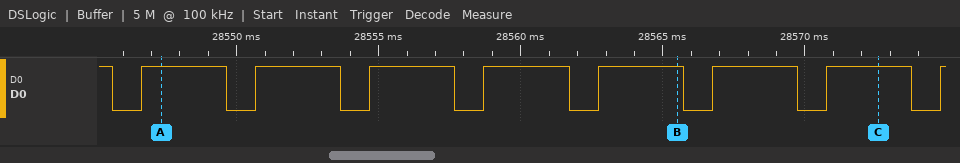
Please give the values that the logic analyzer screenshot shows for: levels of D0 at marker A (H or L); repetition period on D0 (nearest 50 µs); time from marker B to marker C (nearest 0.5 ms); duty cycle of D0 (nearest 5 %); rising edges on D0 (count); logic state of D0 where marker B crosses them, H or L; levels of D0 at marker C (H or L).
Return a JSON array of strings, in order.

["D0=H", "4000 µs", "7 ms", "75 %", "8", "D0=H", "D0=H"]
